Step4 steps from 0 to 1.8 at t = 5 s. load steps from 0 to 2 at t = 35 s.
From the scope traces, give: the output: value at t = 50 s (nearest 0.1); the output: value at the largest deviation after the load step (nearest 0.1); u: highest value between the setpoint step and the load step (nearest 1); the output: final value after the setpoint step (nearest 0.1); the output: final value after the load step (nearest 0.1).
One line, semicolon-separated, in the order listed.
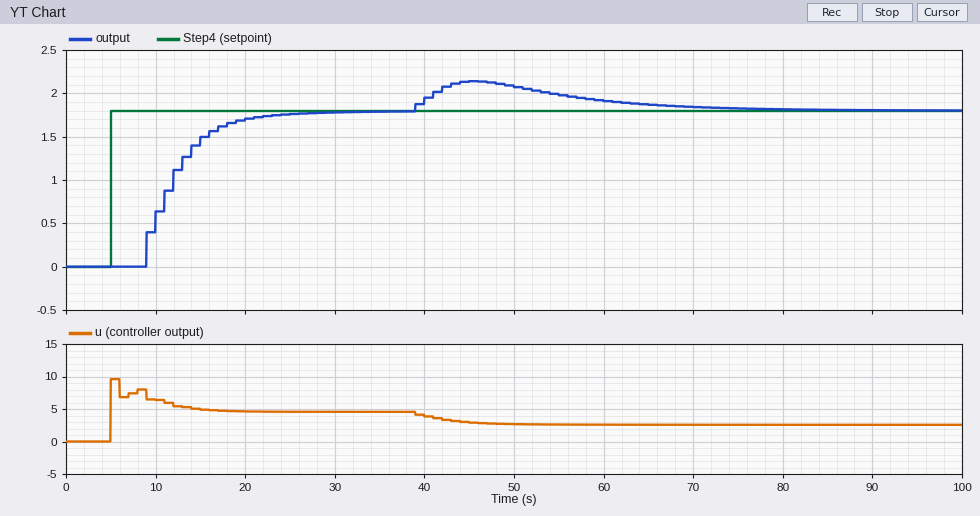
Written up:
2.1; 2.1; 10; 1.8; 1.8
